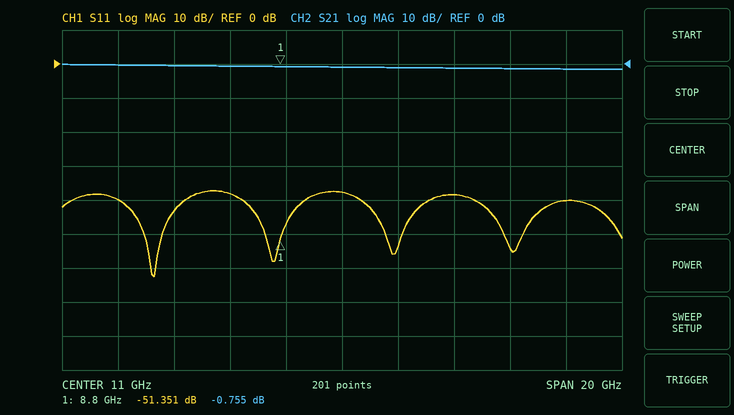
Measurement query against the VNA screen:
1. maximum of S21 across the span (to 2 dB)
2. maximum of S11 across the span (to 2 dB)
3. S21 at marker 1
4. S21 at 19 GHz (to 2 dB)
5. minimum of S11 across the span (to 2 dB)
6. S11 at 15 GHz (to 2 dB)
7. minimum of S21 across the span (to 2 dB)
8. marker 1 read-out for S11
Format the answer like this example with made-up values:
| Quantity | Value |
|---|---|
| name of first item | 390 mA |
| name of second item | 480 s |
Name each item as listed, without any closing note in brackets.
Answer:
| Quantity | Value |
|---|---|
| maximum of S21 across the span | 0 dB |
| maximum of S11 across the span | -38 dB |
| S21 at marker 1 | -0.755 dB |
| S21 at 19 GHz | -2 dB |
| minimum of S11 across the span | -62 dB |
| S11 at 15 GHz | -38 dB |
| minimum of S21 across the span | -2 dB |
| marker 1 read-out for S11 | -51.351 dB |
